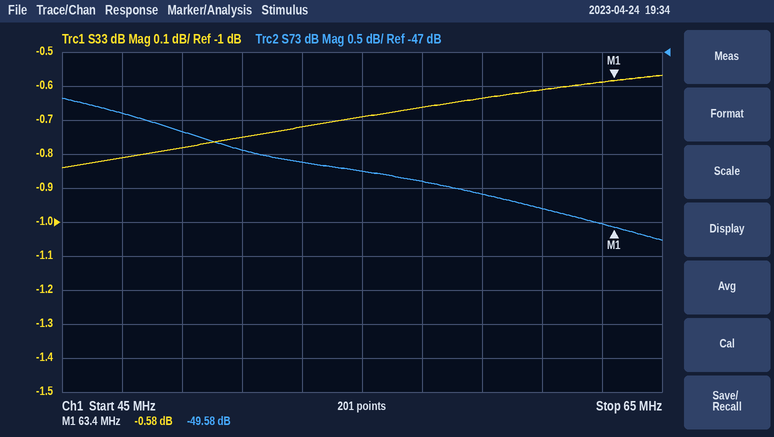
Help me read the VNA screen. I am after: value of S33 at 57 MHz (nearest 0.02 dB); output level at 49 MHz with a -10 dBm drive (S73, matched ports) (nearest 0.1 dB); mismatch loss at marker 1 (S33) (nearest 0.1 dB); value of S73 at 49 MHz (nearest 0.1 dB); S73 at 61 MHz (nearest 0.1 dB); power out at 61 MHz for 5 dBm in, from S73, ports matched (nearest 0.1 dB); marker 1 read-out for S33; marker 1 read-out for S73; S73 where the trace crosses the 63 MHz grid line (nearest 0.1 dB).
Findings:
-0.66 dB
-58.2 dBm
9.0 dB
-48.2 dB
-49.3 dB
-44.3 dBm
-0.58 dB
-49.58 dB
-49.5 dB
